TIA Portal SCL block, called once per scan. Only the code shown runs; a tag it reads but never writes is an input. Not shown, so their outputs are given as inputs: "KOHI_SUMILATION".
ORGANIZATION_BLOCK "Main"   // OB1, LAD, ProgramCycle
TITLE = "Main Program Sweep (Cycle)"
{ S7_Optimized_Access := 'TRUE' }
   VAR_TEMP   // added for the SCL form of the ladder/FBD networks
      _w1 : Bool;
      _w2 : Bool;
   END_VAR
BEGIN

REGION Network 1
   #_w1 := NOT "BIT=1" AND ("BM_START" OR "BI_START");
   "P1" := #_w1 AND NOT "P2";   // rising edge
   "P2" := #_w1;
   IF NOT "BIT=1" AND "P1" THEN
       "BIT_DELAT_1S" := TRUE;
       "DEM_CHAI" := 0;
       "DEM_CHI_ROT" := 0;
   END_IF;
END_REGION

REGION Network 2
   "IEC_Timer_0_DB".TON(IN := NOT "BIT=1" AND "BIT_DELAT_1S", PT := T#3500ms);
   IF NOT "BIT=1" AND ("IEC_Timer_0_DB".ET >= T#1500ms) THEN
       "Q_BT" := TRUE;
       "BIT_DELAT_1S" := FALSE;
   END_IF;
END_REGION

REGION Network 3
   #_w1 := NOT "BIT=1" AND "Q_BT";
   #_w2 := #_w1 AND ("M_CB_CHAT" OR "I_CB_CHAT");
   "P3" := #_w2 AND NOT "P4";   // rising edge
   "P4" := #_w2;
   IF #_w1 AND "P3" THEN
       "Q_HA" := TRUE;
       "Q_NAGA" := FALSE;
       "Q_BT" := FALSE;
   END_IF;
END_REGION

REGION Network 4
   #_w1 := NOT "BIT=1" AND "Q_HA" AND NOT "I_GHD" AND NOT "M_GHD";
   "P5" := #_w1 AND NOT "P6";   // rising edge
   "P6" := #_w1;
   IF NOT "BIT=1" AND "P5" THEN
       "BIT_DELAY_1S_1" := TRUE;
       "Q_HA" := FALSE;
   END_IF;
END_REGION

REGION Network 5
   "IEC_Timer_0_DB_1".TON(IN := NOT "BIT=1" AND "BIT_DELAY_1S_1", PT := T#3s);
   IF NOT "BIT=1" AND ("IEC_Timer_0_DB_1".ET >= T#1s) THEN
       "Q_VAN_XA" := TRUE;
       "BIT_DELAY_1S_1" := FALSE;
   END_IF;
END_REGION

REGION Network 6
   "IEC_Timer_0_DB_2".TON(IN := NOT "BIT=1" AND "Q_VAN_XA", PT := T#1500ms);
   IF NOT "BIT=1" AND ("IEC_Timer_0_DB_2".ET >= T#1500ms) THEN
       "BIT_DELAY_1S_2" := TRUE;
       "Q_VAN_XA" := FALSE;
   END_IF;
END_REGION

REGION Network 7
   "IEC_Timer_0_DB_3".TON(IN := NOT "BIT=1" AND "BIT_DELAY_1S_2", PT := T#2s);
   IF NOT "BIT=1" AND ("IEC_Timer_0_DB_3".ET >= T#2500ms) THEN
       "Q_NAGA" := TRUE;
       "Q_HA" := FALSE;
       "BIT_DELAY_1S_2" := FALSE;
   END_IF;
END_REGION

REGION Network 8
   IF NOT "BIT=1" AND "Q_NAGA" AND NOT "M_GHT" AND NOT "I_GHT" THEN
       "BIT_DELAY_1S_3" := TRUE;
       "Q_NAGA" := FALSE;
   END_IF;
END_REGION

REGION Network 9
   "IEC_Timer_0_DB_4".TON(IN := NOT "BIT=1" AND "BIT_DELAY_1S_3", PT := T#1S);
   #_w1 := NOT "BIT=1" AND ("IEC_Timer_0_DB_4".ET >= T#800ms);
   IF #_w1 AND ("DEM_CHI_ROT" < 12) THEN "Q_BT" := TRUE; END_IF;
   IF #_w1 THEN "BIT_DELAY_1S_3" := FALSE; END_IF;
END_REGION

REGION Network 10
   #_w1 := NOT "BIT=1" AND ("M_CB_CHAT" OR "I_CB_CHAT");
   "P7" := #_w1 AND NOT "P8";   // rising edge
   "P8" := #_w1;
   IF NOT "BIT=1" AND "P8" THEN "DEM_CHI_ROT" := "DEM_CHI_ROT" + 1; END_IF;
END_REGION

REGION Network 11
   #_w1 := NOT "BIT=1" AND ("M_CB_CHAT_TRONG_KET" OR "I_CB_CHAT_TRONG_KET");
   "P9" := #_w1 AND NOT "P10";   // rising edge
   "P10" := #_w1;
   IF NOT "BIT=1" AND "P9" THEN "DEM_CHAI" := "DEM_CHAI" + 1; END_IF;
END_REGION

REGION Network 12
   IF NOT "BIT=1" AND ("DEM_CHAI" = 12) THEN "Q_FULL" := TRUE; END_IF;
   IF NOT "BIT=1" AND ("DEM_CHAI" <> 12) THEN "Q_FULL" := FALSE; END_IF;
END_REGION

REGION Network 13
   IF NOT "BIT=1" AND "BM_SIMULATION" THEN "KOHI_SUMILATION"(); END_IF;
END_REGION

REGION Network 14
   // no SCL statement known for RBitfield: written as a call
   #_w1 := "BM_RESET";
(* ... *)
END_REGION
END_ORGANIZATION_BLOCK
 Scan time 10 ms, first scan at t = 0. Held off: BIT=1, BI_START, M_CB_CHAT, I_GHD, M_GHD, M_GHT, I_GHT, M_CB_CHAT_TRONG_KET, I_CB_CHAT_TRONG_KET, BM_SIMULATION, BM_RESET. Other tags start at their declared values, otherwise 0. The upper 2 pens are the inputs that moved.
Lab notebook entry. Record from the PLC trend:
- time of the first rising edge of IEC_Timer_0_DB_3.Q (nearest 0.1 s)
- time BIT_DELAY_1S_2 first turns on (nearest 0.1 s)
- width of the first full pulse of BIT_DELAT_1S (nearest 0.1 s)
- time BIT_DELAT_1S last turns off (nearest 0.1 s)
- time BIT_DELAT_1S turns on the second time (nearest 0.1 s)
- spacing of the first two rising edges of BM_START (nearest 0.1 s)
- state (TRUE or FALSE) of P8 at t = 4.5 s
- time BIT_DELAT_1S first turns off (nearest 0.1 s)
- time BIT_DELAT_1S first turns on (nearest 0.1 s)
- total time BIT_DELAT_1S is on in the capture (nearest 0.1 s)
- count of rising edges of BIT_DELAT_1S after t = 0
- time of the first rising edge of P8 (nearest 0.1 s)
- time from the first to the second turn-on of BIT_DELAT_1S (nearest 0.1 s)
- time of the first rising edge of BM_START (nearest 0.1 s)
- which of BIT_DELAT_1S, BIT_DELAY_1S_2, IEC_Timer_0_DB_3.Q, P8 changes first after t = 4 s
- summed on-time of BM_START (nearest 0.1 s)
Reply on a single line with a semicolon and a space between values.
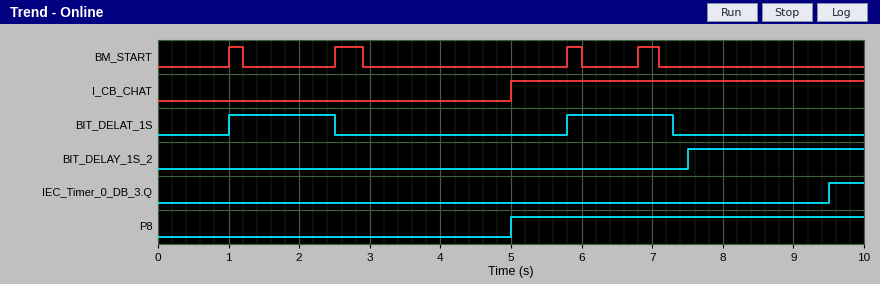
9.5 s; 7.5 s; 1.5 s; 7.3 s; 5.8 s; 1.5 s; FALSE; 2.5 s; 1.0 s; 3.0 s; 2; 5.0 s; 4.8 s; 1.0 s; P8; 1.1 s
